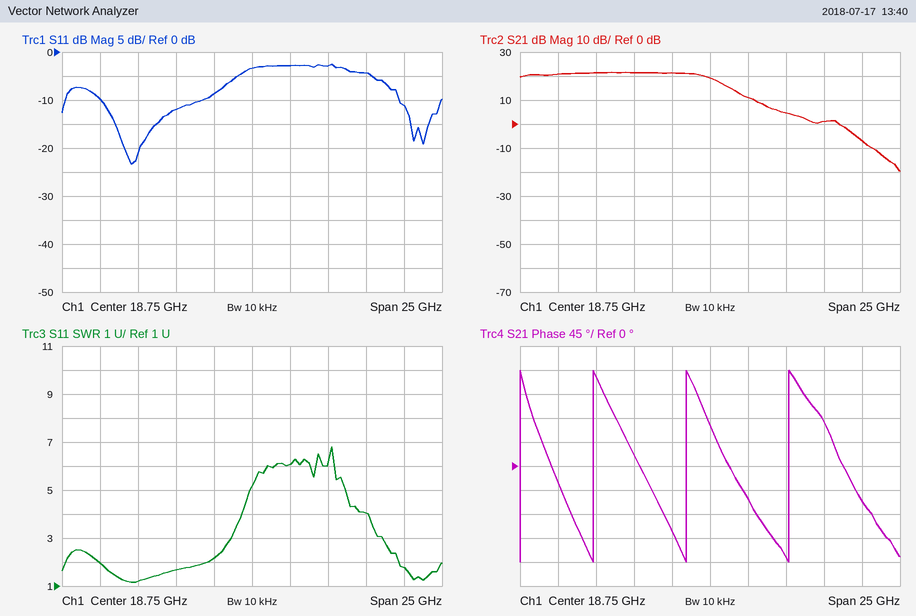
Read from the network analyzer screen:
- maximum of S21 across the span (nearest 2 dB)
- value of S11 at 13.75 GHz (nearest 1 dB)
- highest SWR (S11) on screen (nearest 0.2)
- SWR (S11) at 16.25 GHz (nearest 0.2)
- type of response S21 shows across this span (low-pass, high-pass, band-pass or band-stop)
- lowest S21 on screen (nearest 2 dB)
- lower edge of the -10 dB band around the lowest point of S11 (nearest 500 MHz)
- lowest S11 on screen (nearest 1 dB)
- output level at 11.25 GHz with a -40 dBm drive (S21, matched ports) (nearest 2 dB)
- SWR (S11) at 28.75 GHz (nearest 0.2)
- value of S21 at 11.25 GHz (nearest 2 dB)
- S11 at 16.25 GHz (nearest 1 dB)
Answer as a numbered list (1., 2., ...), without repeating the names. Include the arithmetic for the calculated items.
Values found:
1. 22 dB
2. -12 dB
3. 6.8
4. 2.2
5. low-pass
6. -20 dB
7. 9.0 GHz
8. -23 dB
9. -40 dBm + (22 dB) = -18 dBm
10. 1.8
11. 22 dB
12. -9 dB
